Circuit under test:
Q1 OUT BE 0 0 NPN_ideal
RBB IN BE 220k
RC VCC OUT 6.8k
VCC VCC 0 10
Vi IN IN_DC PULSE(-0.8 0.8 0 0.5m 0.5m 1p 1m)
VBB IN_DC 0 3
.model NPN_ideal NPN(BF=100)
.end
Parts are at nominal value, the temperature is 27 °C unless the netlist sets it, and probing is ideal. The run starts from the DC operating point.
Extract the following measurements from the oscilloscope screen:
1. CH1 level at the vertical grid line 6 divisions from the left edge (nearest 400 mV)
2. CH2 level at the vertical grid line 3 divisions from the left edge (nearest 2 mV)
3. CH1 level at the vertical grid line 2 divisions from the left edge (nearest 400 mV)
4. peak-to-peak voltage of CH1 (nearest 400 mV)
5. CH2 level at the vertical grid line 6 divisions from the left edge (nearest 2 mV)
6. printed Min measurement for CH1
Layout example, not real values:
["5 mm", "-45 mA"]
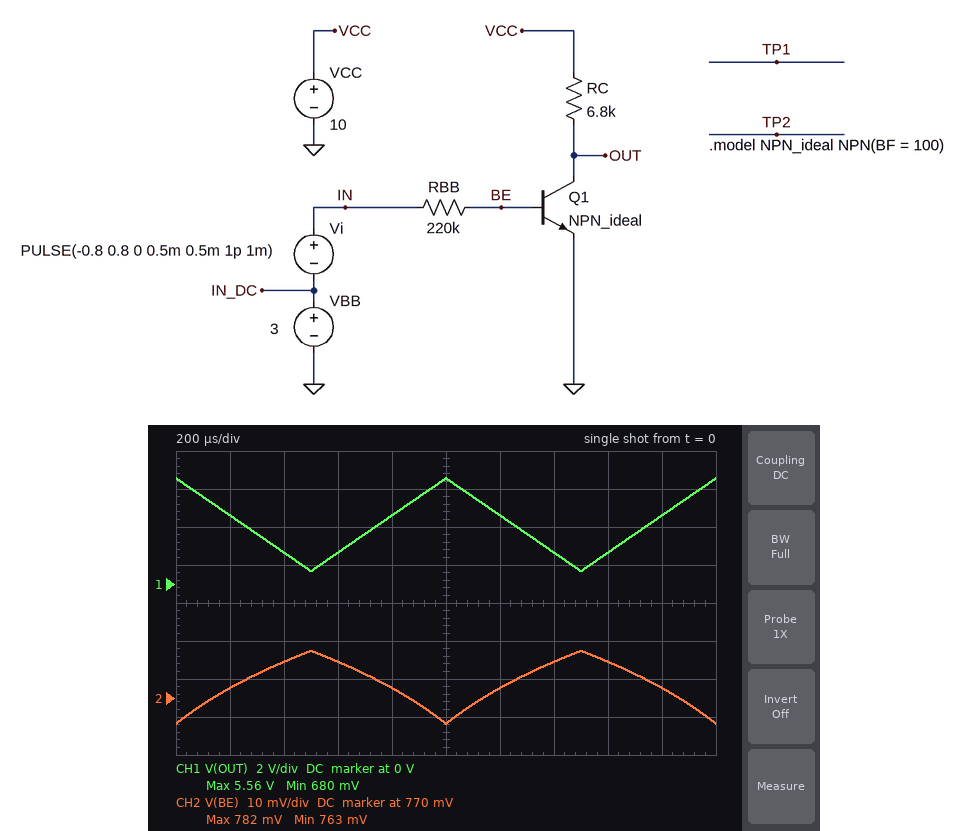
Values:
["3.6 V", "780 mV", "1.6 V", "4.8 V", "772 mV", "680 mV"]
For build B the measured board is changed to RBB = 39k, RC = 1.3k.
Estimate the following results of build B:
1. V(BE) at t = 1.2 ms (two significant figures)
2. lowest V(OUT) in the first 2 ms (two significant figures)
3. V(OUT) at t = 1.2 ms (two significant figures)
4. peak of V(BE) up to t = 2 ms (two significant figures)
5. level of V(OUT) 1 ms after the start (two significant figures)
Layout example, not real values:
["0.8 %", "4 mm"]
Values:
["820 mV", "230 mV", "3.3 V", "830 mV", "5.4 V"]
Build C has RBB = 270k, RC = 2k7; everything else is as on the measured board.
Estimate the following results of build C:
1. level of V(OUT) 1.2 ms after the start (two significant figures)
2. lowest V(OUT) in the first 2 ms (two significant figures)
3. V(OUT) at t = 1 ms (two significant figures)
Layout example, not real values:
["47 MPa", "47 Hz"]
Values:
["7.9 V", "7.0 V", "8.6 V"]
